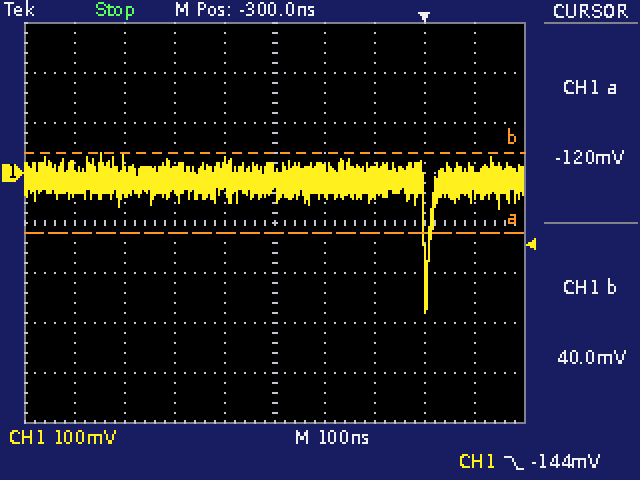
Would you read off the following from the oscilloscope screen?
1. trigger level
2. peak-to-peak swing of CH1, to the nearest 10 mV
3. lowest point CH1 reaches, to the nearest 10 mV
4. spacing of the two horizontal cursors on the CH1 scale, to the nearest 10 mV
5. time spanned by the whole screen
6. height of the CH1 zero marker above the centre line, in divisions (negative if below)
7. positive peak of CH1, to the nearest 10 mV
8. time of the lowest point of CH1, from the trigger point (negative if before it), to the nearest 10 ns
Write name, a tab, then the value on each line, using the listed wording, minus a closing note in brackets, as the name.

trigger level	-144 mV
peak-to-peak swing of CH1, to the nearest 10 mV	320 mV
lowest point CH1 reaches, to the nearest 10 mV	-280 mV
spacing of the two horizontal cursors on the CH1 scale, to the nearest 10 mV	160 mV
time spanned by the whole screen	1 µs
height of the CH1 zero marker above the centre line, in divisions	+1.0 div
positive peak of CH1, to the nearest 10 mV	40 mV
time of the lowest point of CH1, from the trigger point (negative if before it), to the nearest 10 ns	0 ns
